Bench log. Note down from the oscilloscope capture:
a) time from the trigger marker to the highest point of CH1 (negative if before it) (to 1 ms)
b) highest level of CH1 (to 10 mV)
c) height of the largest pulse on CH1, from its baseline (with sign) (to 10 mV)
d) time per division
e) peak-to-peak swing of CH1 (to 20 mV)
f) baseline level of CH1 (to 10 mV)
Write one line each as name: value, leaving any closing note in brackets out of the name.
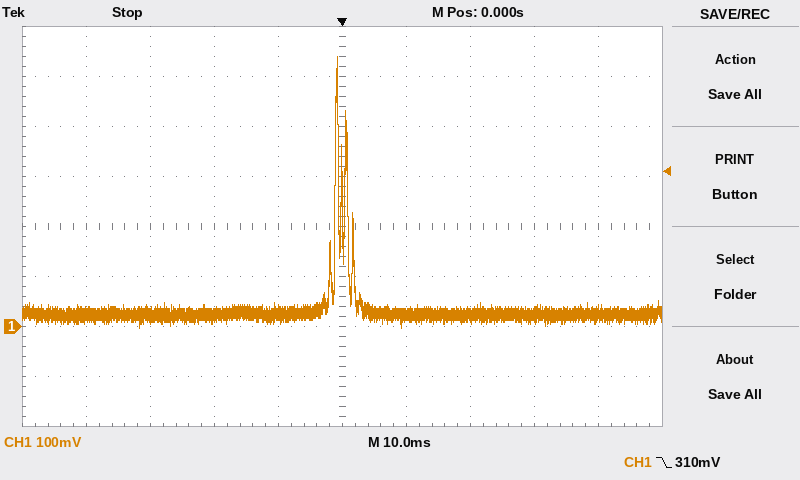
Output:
time from the trigger marker to the highest point of CH1 (negative if before it): -1 ms
highest level of CH1: 540 mV
height of the largest pulse on CH1, from its baseline (with sign): +520 mV
time per division: 10 ms
peak-to-peak swing of CH1: 540 mV
baseline level of CH1: 20 mV
